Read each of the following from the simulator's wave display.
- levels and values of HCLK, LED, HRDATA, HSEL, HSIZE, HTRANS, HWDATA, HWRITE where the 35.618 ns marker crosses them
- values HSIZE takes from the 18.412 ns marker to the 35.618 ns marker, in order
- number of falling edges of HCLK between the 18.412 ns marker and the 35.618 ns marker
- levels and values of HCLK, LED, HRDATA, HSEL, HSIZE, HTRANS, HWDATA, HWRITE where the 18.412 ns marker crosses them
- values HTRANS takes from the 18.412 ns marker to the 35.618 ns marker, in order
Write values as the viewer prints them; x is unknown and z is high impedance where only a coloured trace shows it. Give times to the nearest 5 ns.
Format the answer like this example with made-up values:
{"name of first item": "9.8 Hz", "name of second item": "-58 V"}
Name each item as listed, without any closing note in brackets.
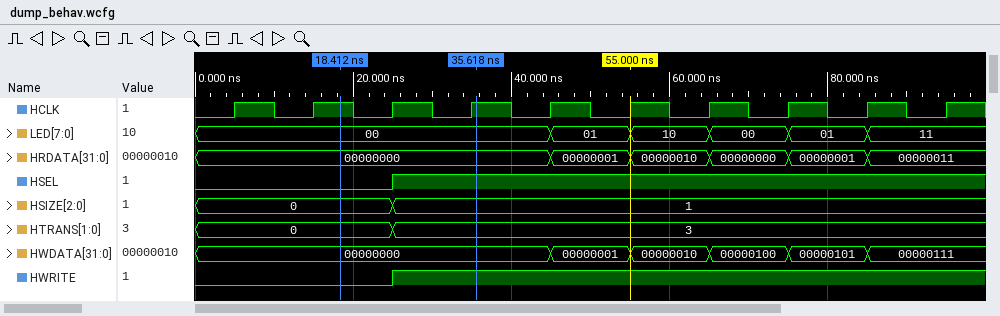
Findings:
{"levels and values of HCLK, LED, HRDATA, HSEL, HSIZE, HTRANS, HWDATA, HWRITE where the 35.618 ns marker crosses them": "HCLK=1, LED=00, HRDATA=00000000, HSEL=1, HSIZE=1, HTRANS=3, HWDATA=00000000, HWRITE=1", "values HSIZE takes from the 18.412 ns marker to the 35.618 ns marker, in order": "0, 1", "number of falling edges of HCLK between the 18.412 ns marker and the 35.618 ns marker": "2", "levels and values of HCLK, LED, HRDATA, HSEL, HSIZE, HTRANS, HWDATA, HWRITE where the 18.412 ns marker crosses them": "HCLK=1, LED=00, HRDATA=00000000, HSEL=0, HSIZE=0, HTRANS=0, HWDATA=00000000, HWRITE=0", "values HTRANS takes from the 18.412 ns marker to the 35.618 ns marker, in order": "0, 3"}
